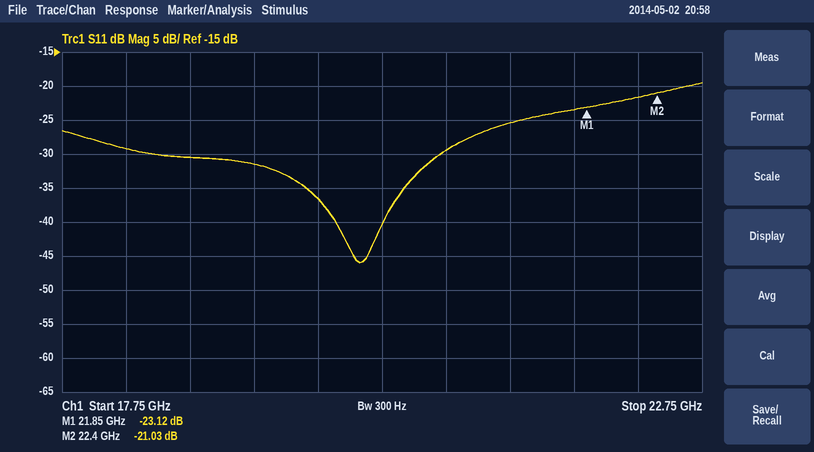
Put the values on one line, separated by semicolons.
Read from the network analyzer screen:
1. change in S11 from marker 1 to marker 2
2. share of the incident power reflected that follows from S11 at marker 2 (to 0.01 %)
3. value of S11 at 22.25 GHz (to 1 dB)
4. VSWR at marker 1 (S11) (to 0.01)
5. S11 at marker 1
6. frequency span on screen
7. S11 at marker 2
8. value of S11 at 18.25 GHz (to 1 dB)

2.09 dB; 0.79 %; -22 dB; 1.15; -23.12 dB; 5 GHz; -21.03 dB; -29 dB
